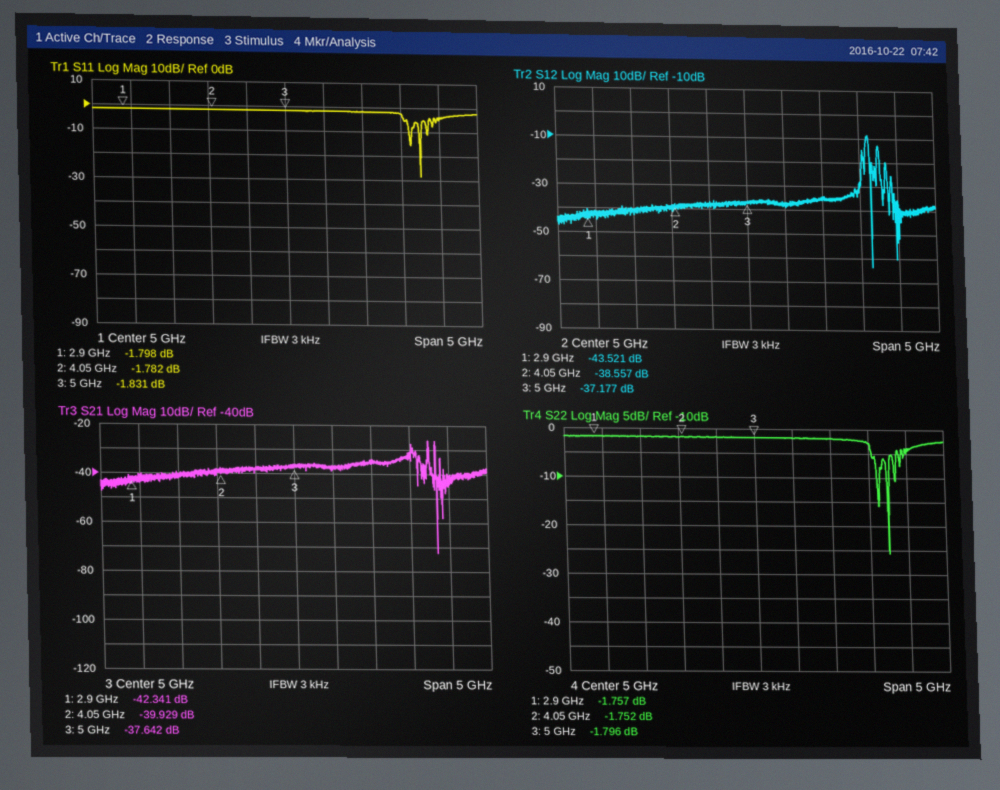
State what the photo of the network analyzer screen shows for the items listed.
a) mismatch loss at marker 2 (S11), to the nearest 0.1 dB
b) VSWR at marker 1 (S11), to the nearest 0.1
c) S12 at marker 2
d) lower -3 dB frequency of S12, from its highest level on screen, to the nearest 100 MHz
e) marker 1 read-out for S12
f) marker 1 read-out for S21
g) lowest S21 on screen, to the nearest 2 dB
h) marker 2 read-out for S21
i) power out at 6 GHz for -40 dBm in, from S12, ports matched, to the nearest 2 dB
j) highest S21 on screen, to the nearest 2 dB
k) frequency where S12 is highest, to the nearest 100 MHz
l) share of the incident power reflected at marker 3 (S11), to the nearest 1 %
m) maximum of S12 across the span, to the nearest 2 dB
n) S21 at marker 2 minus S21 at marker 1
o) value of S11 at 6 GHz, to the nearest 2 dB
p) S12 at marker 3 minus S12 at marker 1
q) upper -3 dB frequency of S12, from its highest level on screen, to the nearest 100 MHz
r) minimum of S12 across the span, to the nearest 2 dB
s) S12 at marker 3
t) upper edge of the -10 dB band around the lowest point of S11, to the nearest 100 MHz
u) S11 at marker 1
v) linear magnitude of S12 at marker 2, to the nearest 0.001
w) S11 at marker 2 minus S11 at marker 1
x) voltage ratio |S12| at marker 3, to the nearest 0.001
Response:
4.7 dB
9.7
-38.557 dB
6.6 GHz
-43.521 dB
-42.341 dB
-72 dB
-39.929 dB
-76 dBm
-26 dB
6.6 GHz
66 %
-8 dB
2.412 dB
-2 dB
6.344 dB
6.6 GHz
-64 dB
-37.177 dB
6.8 GHz
-1.798 dB
0.012
0.016 dB
0.014
